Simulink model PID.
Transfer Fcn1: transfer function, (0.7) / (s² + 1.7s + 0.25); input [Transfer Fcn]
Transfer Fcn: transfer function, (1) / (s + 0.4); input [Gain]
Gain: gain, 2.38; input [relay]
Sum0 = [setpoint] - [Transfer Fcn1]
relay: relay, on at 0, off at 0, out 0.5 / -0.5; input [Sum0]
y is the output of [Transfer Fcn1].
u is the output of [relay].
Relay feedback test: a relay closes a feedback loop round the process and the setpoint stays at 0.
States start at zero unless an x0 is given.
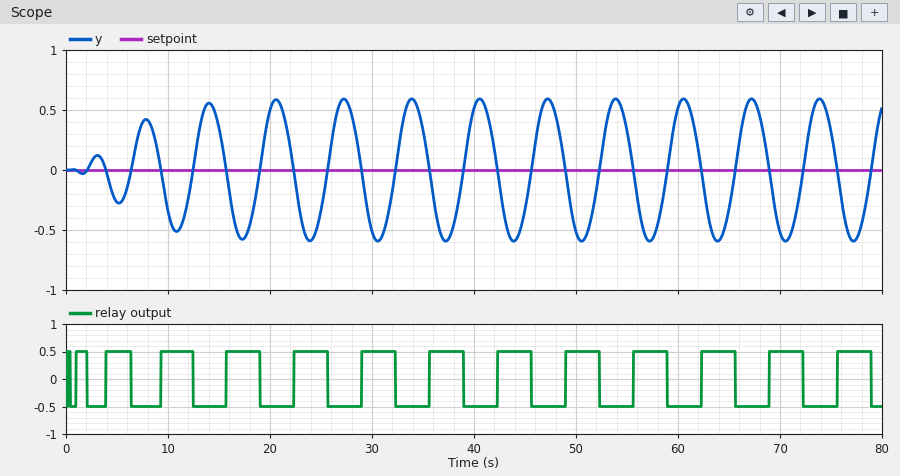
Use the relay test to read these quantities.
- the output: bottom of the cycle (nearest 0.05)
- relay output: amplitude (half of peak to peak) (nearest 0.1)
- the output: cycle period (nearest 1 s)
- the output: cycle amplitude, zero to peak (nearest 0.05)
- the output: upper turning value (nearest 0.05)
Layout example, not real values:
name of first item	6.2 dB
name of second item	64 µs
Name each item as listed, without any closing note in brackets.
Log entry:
the output: bottom of the cycle	-0.60
relay output: amplitude (half of peak to peak)	0.5
the output: cycle period	7 s
the output: cycle amplitude, zero to peak	0.60
the output: upper turning value	0.60
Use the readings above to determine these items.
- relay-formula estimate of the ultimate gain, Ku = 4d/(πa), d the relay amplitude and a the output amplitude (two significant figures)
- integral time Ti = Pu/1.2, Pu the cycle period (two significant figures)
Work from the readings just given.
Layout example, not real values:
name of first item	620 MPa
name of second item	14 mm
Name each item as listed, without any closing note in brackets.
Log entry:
relay-formula estimate of the ultimate gain, Ku = 4d/(πa), d the relay amplitude and a the output amplitude	1.1
integral time Ti = Pu/1.2, Pu the cycle period	5.8 s
